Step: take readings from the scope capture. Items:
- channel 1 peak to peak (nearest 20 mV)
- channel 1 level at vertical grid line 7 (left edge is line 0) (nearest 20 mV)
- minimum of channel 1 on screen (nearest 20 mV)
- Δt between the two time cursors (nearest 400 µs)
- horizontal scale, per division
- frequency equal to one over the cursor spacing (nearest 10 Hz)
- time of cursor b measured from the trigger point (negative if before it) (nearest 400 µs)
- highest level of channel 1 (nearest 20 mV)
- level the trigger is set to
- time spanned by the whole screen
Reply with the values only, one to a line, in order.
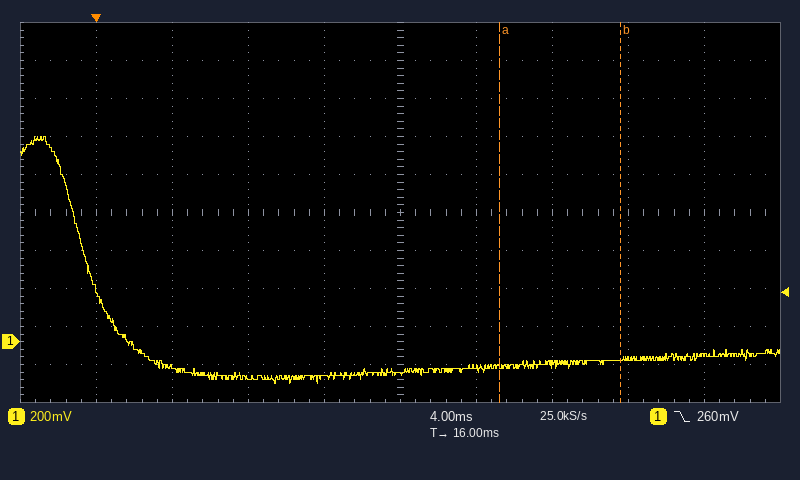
1.30 V
-120 mV
-220 mV
6.4 ms
4 ms
160 Hz
+27.6 ms
1.08 V
260 mV
40 ms
